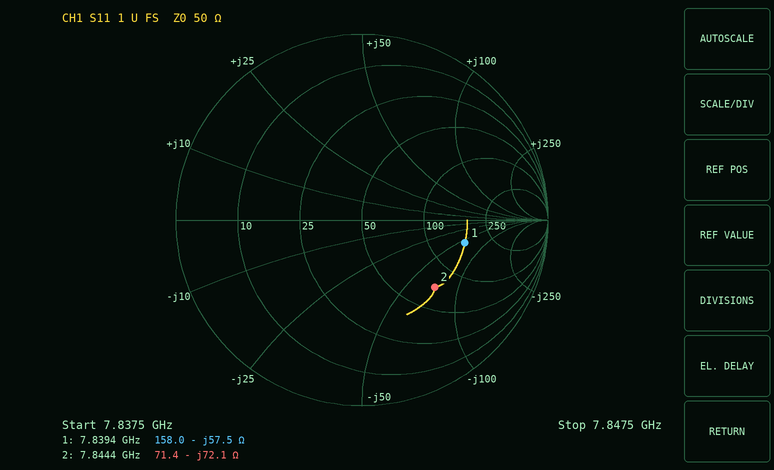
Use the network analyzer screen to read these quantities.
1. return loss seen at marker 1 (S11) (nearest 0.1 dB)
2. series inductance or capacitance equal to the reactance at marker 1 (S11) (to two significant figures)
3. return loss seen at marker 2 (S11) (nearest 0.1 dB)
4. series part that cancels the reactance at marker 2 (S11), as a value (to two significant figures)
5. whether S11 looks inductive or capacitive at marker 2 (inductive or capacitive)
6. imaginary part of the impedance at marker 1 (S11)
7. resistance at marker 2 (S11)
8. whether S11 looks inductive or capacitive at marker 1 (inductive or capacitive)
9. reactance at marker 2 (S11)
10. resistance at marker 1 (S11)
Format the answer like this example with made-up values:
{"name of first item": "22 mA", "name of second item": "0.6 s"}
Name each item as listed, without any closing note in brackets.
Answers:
{"return loss seen at marker 1 (S11)": "4.9 dB", "series inductance or capacitance equal to the reactance at marker 1 (S11)": "350 fF", "return loss seen at marker 2 (S11)": "5.5 dB", "series part that cancels the reactance at marker 2 (S11), as a value": "1.5 nH", "whether S11 looks inductive or capacitive at marker 2": "capacitive", "imaginary part of the impedance at marker 1": "-57.5 Ω", "resistance at marker 2": "71.4 Ω", "whether S11 looks inductive or capacitive at marker 1": "capacitive", "reactance at marker 2": "-72.1 Ω", "resistance at marker 1": "158.0 Ω"}
